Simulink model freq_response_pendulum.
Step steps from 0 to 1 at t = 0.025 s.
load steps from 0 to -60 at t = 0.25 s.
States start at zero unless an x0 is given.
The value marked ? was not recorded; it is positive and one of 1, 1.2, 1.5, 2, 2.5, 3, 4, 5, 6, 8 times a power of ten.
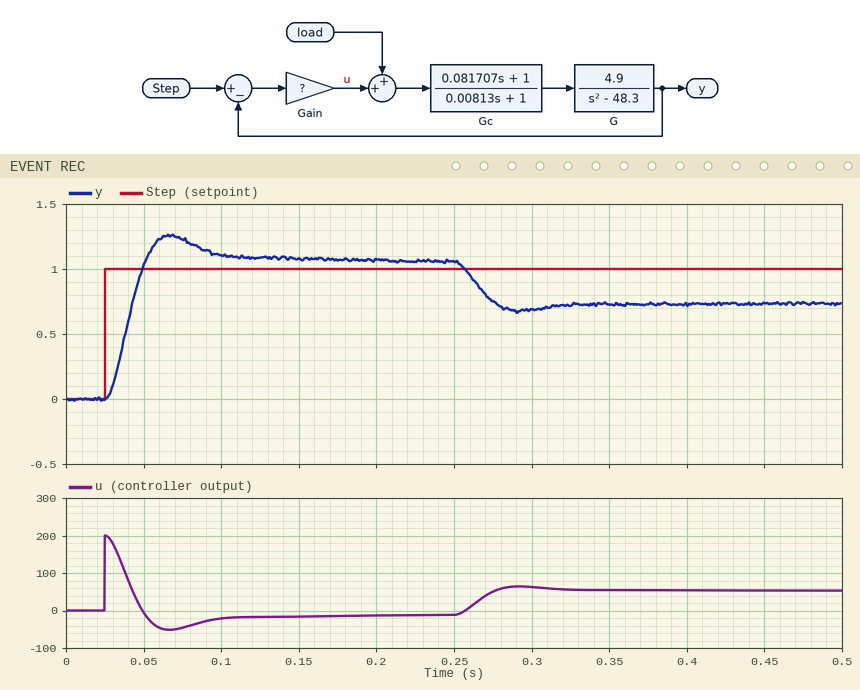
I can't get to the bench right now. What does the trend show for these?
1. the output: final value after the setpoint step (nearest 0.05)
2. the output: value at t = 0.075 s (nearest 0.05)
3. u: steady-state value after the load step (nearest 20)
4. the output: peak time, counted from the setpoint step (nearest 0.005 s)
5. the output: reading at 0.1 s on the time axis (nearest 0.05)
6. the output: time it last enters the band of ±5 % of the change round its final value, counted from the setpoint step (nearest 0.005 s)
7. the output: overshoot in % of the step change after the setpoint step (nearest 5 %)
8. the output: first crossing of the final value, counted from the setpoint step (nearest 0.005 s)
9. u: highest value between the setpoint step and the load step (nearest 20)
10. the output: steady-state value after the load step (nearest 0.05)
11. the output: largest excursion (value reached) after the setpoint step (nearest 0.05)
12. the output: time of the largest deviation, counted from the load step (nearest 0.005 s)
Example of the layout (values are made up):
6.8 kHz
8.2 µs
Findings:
1.05
1.25
60
0.040 s
1.10
0.075 s
20 %
0.025 s
200
0.75
1.25
0.040 s
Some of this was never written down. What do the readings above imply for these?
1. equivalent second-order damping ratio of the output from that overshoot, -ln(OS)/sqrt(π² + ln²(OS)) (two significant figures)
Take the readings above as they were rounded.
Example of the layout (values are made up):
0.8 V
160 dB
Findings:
0.46
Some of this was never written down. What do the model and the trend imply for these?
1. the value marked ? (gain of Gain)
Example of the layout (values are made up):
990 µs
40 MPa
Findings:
200
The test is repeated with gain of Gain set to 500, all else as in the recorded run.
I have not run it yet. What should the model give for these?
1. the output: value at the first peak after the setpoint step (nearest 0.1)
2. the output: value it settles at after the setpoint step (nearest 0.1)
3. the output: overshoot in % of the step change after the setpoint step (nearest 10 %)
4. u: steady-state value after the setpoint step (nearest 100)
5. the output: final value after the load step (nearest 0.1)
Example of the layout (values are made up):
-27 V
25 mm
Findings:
1.4
1.0
30 %
0
0.9
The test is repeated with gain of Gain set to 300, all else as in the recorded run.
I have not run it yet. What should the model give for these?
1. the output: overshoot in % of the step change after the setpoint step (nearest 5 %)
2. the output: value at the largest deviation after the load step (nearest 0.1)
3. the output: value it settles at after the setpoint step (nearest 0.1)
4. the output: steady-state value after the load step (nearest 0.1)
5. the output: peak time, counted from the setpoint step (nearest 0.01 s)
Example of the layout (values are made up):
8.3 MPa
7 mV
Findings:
25 %
0.8
1.0
0.8
0.03 s
